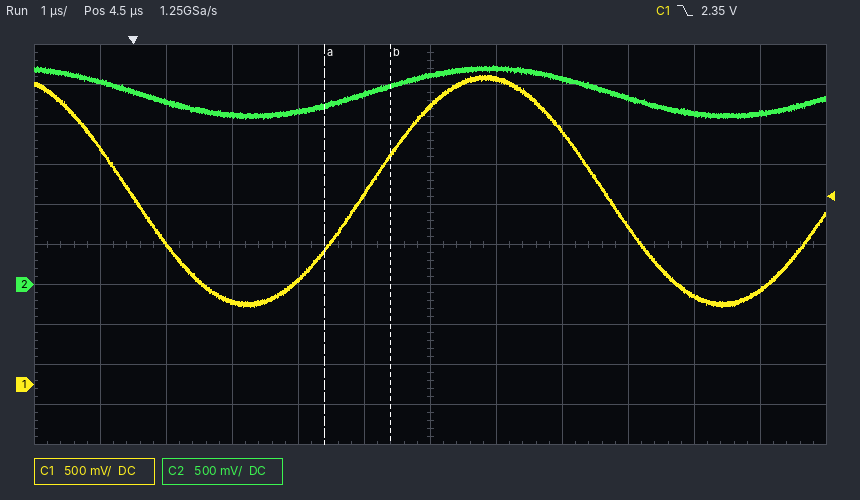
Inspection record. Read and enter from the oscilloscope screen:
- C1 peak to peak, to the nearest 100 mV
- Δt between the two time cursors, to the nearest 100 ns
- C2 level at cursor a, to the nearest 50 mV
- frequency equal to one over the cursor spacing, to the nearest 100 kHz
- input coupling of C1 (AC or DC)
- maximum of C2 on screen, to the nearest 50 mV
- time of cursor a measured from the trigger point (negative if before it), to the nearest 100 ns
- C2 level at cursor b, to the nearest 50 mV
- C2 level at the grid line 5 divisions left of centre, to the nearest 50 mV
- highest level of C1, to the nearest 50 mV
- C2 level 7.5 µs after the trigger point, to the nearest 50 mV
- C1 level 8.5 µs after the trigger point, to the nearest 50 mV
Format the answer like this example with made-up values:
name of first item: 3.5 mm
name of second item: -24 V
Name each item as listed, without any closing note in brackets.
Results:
C1 peak to peak, to the nearest 100 mV: 2.90 V
Δt between the two time cursors, to the nearest 100 ns: 1.0 µs
C2 level at cursor a, to the nearest 50 mV: 2.25 V
frequency equal to one over the cursor spacing, to the nearest 100 kHz: 1.0 MHz
input coupling of C1: DC
maximum of C2 on screen, to the nearest 50 mV: 2.75 V
time of cursor a measured from the trigger point (negative if before it), to the nearest 100 ns: +2.9 µs
C2 level at cursor b, to the nearest 50 mV: 2.50 V
C2 level at the grid line 5 divisions left of centre, to the nearest 50 mV: 2.55 V
highest level of C1, to the nearest 50 mV: 3.85 V
C2 level 7.5 µs after the trigger point, to the nearest 50 mV: 2.35 V
C1 level 8.5 µs after the trigger point, to the nearest 50 mV: 1.10 V
